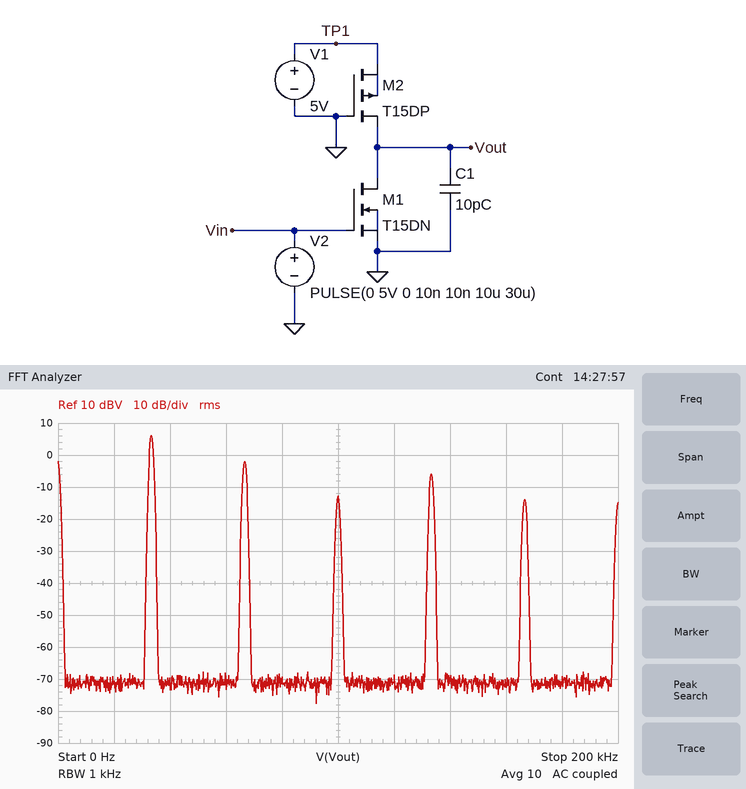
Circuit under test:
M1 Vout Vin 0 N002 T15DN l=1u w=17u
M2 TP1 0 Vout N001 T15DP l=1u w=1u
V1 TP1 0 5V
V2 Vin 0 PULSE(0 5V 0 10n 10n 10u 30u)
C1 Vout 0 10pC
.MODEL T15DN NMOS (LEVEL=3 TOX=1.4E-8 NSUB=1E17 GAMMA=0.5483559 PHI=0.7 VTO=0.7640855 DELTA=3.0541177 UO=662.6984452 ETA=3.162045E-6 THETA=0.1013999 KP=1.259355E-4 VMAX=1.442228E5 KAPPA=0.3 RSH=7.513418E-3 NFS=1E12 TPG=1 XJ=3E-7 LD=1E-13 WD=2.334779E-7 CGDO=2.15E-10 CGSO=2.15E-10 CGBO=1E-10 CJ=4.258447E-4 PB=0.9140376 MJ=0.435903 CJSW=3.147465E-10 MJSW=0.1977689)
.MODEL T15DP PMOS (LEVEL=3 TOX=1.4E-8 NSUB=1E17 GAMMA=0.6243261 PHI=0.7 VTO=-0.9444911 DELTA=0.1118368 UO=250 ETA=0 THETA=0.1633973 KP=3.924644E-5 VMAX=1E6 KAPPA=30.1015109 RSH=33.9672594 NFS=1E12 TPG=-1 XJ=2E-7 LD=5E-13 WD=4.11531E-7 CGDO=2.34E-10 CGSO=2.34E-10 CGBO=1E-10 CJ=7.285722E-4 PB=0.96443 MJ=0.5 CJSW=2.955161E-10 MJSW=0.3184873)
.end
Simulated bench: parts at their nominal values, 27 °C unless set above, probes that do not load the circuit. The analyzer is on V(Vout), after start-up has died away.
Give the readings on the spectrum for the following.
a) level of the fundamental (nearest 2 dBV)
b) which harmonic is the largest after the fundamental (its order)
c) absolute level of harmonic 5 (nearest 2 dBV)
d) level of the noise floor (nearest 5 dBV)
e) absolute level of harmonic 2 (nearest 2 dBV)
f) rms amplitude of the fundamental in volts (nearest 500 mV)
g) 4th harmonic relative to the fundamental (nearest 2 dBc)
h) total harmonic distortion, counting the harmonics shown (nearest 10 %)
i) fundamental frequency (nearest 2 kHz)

6 dBV
2
-14 dBV
-70 dBV
-2 dBV
2.0 V
-12 dBc
50 %
34 kHz
